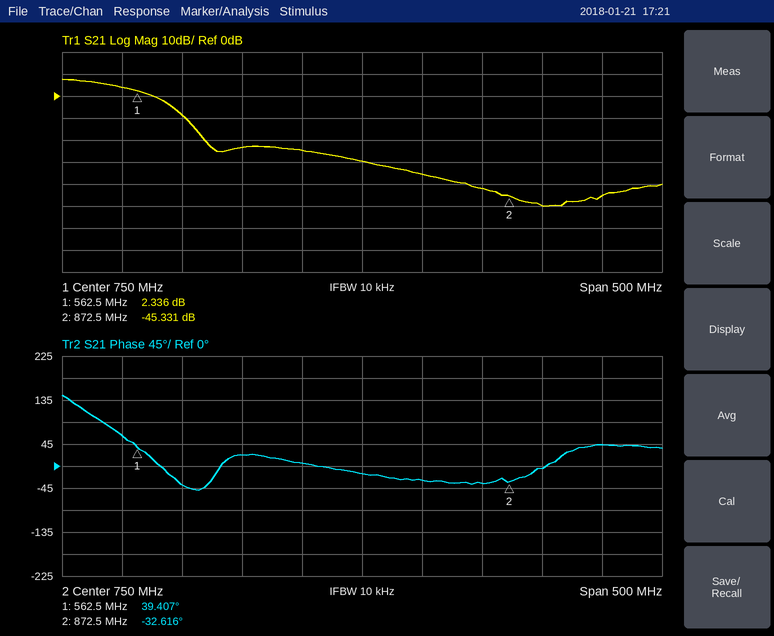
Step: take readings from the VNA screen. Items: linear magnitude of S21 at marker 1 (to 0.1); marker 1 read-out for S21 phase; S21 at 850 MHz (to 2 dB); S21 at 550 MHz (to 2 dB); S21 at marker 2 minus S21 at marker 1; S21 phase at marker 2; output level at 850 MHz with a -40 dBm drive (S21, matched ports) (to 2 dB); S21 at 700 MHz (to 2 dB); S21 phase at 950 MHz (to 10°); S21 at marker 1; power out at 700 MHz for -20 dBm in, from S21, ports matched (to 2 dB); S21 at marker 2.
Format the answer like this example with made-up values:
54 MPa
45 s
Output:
1.3
39.407°
-42 dB
4 dB
-47.667 dB
-32.616°
-82 dBm
-24 dB
40°
2.336 dB
-44 dBm
-45.331 dB
